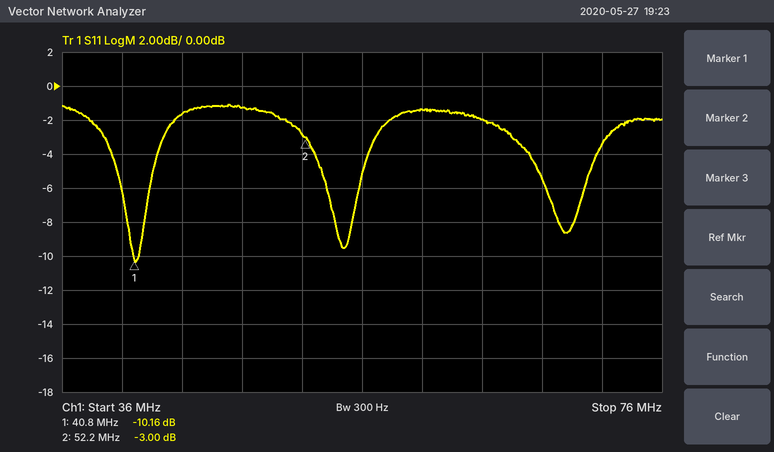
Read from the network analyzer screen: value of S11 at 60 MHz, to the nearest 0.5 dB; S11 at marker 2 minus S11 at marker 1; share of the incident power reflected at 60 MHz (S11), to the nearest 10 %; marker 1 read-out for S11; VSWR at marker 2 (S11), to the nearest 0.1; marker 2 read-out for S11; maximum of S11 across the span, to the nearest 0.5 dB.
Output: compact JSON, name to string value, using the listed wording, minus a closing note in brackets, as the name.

{"value of S11 at 60 MHz, to the nearest 0.5 dB": "-1.5 dB", "S11 at marker 2 minus S11 at marker 1": "7.16 dB", "share of the incident power reflected at 60 MHz (S11), to the nearest 10 %": "70 %", "marker 1 read-out for S11": "-10.16 dB", "VSWR at marker 2 (S11), to the nearest 0.1": "5.8", "marker 2 read-out for S11": "-3.00 dB", "maximum of S11 across the span, to the nearest 0.5 dB": "-1.0 dB"}
